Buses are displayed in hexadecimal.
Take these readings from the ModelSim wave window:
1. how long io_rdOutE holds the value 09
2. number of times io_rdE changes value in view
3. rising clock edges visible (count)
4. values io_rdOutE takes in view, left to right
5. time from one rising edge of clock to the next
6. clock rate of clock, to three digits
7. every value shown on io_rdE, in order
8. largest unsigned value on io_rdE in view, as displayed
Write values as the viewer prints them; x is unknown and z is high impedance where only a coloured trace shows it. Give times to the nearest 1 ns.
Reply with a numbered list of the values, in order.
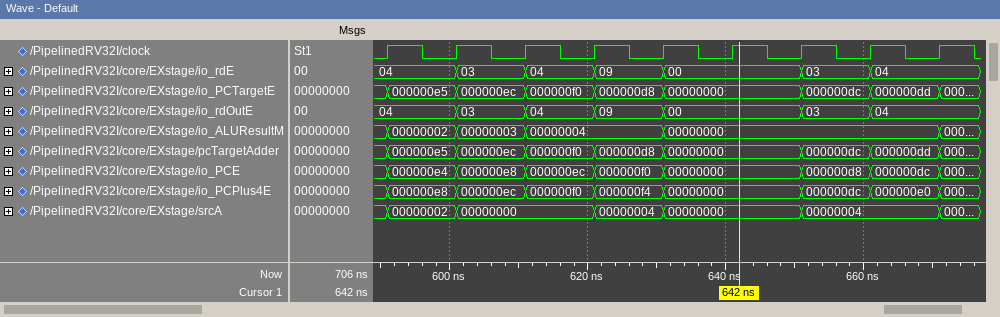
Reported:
1. 10 ns
2. 6
3. 9
4. 04, 03, 04, 09, 00, 03, 04
5. 10 ns
6. 100 MHz
7. 04, 03, 04, 09, 00, 03, 04
8. 09
